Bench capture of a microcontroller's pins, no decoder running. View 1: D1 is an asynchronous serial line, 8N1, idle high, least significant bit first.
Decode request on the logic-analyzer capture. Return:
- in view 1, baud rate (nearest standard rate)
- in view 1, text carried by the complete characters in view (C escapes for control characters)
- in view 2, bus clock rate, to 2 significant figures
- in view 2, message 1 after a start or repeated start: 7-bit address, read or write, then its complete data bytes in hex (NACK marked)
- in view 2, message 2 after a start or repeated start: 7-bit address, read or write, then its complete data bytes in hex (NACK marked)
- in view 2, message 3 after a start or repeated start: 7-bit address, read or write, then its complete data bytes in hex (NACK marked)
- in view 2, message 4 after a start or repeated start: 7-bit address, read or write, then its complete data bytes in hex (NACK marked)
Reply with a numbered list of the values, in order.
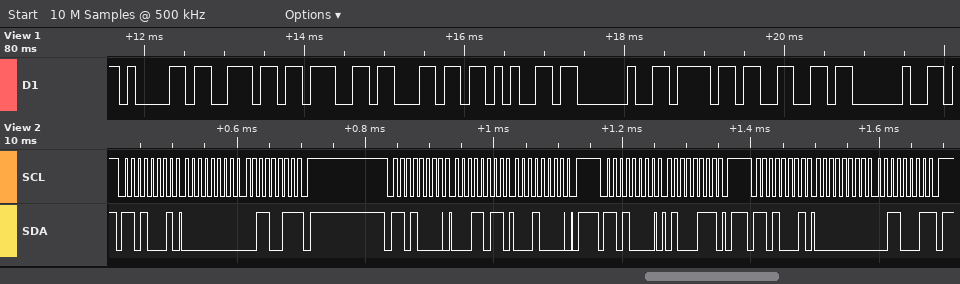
1. 9600 baud
2. "angle of "
3. 100 kHz
4. 0x68 read: 00 33 NACK
5. 0x68 write: 1B 10
6. 0x68 write: 47
7. 0x68 read: 00 31 NACK
